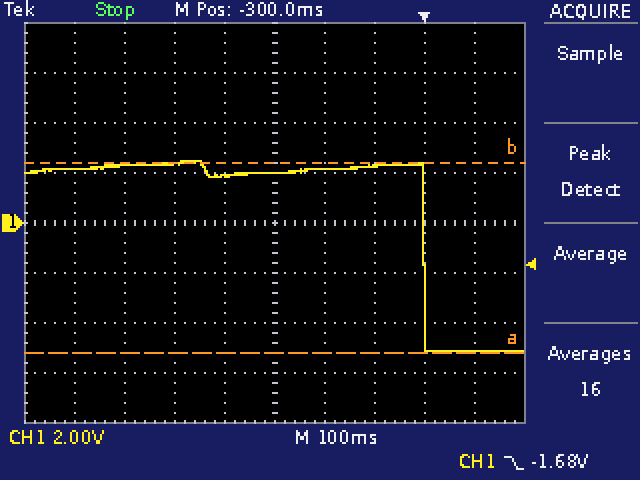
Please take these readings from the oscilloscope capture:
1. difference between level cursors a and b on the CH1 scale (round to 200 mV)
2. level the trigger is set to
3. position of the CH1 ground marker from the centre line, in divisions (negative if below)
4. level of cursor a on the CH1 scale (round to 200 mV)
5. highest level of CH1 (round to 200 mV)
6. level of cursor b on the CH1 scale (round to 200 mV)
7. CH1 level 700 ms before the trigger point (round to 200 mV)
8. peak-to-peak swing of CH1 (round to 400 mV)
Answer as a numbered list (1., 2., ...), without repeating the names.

1. 7.6 V
2. -1.68 V
3. 0.0 div
4. -5.2 V
5. 2.4 V
6. 2.4 V
7. 2.2 V
8. 7.6 V
